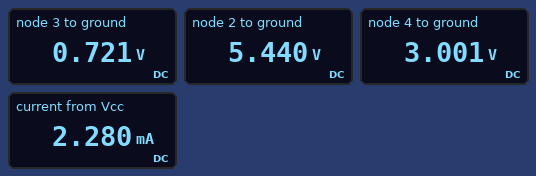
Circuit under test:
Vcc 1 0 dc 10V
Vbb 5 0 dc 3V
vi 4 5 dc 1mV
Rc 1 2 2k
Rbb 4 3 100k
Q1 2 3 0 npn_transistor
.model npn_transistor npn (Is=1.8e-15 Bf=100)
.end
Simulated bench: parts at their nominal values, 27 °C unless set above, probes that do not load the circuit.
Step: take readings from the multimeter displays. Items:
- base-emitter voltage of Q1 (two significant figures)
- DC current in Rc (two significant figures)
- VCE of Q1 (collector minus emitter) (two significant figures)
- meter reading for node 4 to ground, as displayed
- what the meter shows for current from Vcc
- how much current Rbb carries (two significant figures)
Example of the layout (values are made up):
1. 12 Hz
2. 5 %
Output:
1. 720 mV
2. 2.3 mA
3. 5.4 V
4. 3.001 V
5. 2.280 mA
6. 23 µA
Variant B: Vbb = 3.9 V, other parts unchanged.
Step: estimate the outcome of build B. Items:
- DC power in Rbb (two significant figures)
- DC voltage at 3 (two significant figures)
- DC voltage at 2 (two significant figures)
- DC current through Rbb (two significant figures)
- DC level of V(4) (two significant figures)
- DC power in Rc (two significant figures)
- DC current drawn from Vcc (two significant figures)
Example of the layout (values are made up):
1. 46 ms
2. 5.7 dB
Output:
1. 100 µW
2. 730 mV
3. 3.7 V
4. 32 µA
5. 3.9 V
6. 20 mW
7. 3.2 mA
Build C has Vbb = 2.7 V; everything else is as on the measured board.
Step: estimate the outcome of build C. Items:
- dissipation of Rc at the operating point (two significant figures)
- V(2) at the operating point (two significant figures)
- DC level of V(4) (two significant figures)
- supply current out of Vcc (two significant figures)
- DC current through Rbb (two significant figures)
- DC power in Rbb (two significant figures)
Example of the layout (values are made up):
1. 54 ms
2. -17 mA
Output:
1. 7.9 mW
2. 6.0 V
3. 2.7 V
4. 2.0 mA
5. 20 µA
6. 39 µW
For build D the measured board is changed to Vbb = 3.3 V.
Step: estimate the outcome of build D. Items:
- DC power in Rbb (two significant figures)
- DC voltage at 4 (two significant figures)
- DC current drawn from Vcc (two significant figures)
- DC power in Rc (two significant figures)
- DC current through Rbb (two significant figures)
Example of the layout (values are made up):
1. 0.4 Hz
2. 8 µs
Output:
1. 66 µW
2. 3.3 V
3. 2.6 mA
4. 13 mW
5. 26 µA
